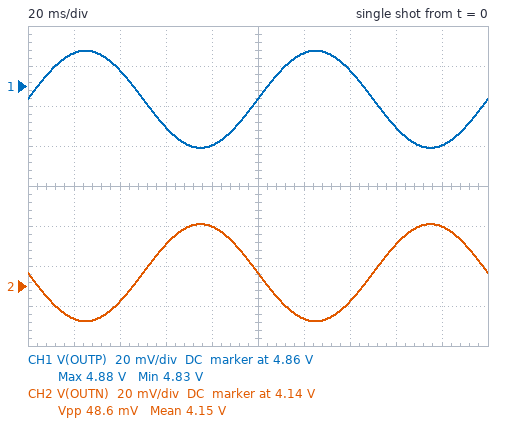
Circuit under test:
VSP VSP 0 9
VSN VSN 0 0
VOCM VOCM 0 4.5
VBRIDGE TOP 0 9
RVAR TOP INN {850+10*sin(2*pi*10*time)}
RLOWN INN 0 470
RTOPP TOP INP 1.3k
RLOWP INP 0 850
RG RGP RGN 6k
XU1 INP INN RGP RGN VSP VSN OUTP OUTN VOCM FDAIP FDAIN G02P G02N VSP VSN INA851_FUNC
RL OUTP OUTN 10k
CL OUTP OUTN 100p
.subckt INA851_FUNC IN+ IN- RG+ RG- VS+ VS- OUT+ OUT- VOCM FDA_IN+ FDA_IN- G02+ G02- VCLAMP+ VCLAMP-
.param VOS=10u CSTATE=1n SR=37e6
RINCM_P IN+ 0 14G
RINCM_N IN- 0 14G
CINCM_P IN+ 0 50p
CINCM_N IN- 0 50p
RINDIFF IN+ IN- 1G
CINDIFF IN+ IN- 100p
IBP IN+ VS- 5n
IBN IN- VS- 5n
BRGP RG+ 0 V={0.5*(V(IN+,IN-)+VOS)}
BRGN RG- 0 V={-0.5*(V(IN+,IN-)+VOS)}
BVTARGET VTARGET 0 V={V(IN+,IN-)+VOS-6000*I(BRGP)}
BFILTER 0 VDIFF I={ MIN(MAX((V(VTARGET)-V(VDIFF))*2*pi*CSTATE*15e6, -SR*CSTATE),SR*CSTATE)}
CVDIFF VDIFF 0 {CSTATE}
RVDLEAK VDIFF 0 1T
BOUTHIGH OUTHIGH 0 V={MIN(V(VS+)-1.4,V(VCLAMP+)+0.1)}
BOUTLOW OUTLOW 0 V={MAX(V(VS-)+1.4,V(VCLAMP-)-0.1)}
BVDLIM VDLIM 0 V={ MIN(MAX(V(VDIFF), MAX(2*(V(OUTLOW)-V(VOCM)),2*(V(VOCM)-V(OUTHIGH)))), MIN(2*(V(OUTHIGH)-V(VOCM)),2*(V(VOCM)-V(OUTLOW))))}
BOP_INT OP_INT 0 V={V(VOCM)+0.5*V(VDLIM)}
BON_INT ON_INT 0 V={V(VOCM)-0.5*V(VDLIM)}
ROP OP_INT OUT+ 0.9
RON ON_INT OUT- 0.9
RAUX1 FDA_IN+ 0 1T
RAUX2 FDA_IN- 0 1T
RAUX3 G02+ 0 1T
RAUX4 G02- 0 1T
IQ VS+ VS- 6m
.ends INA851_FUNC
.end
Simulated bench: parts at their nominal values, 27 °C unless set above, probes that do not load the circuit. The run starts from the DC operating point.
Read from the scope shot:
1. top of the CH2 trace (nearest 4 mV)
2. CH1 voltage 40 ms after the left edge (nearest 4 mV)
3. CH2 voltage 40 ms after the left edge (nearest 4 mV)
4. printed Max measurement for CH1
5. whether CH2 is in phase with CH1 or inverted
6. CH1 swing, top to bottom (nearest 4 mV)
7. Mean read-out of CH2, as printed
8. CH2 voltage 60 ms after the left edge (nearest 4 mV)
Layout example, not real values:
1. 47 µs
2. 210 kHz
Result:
1. 4.172 V
2. 4.868 V
3. 4.132 V
4. 4.88 V
5. inverted
6. 48 mV
7. 4.15 V
8. 4.160 V
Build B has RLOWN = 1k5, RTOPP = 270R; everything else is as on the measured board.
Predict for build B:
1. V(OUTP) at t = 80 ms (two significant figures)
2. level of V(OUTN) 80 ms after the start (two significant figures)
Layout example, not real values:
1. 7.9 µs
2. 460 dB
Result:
1. 5.6 V
2. 3.4 V
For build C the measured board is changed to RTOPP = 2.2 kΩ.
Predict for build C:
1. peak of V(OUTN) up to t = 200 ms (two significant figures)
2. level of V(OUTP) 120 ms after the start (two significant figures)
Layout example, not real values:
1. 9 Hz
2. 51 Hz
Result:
1. 5.2 V
2. 3.8 V
